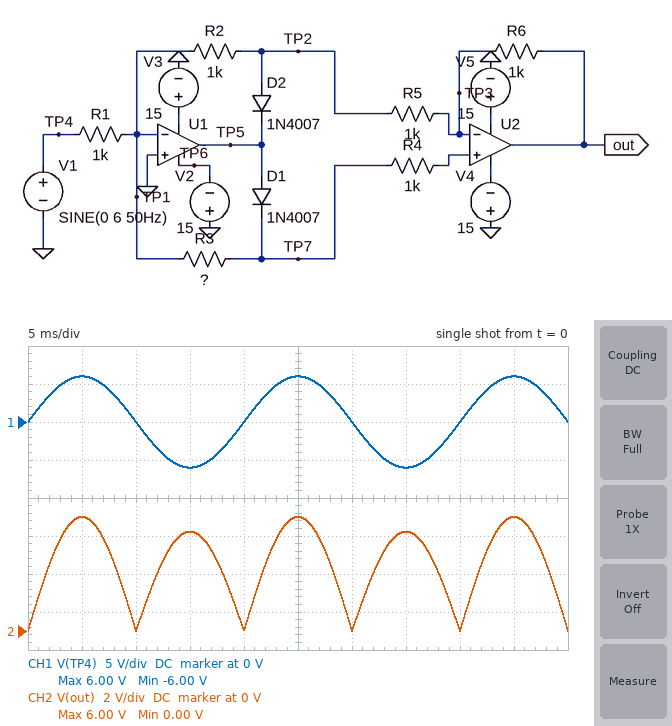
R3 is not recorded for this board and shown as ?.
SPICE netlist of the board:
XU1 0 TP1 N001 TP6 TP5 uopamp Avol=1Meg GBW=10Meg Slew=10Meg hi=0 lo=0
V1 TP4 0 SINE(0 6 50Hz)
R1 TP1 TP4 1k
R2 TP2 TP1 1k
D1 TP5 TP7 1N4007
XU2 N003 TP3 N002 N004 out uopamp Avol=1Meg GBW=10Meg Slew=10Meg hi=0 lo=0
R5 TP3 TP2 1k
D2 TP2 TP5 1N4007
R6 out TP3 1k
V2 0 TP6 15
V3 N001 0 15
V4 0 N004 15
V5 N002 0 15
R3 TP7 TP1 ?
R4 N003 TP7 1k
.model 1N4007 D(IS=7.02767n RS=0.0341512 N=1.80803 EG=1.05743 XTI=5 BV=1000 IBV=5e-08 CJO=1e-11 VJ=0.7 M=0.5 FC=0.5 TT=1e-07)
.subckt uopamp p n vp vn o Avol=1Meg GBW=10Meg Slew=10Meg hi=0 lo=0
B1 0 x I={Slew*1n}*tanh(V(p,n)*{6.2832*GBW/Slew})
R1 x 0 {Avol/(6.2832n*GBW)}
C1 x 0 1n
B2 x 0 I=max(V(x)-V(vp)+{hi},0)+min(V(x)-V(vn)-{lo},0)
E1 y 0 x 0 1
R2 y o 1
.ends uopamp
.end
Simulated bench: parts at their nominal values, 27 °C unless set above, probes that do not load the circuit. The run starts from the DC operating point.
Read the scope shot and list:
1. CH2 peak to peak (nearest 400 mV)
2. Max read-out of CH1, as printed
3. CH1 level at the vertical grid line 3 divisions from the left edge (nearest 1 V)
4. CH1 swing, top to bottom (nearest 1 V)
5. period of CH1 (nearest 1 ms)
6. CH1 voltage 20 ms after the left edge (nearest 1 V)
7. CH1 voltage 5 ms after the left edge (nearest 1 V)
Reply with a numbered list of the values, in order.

1. 6.0 V
2. 6.00 V
3. -6 V
4. 12 V
5. 20 ms
6. 0 V
7. 6 V
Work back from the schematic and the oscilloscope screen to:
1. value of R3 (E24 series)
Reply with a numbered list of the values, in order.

1. 820 Ω
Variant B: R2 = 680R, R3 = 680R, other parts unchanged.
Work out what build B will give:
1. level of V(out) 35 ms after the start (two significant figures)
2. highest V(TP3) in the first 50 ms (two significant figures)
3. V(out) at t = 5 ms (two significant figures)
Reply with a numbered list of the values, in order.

1. 4.6 V
2. 2.9 V
3. 4.1 V
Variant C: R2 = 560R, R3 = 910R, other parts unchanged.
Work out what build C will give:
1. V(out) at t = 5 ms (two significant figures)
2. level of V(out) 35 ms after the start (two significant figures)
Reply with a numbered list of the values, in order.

1. 3.4 V
2. 5.7 V
